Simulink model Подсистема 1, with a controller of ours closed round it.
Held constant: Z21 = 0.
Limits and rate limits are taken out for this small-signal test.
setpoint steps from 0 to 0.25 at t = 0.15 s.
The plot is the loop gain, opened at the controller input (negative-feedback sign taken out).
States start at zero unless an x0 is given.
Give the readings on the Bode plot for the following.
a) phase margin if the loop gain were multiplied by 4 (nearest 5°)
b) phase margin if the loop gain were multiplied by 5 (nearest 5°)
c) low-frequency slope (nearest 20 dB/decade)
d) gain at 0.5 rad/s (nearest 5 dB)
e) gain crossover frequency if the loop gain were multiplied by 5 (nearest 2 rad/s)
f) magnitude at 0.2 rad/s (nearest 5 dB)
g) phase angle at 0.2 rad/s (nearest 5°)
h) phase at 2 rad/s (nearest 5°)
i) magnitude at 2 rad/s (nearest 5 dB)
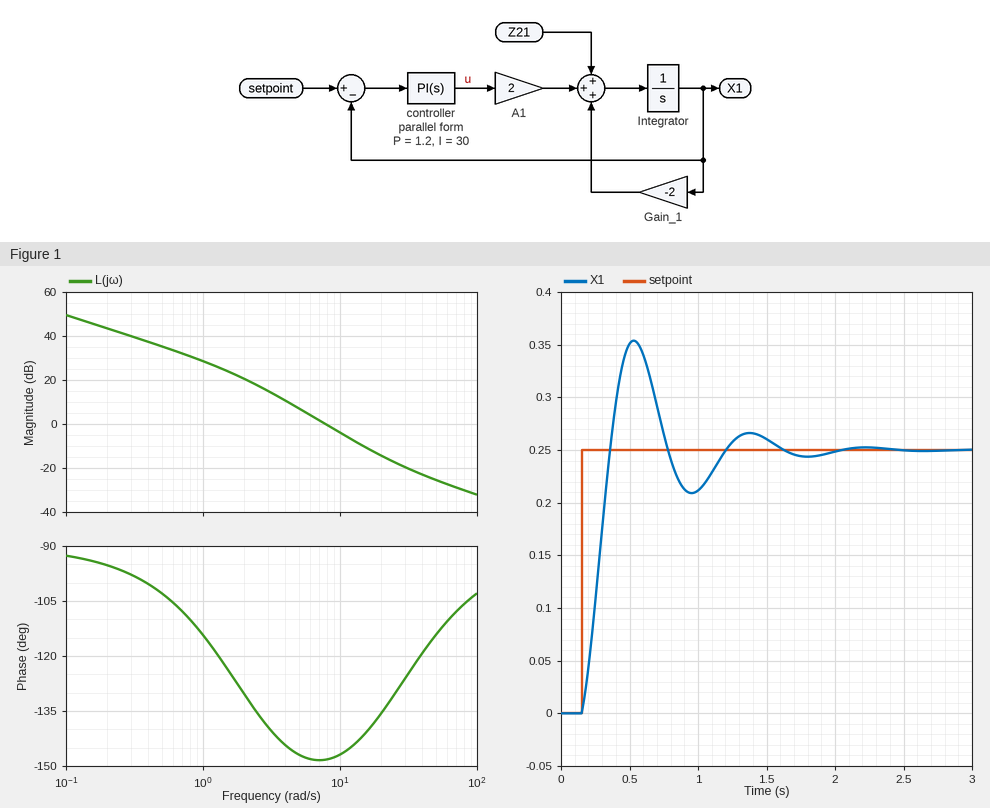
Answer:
40°
45°
-20 dB/decade
35 dB
20 rad/s
45 dB
-95°
-130°
20 dB
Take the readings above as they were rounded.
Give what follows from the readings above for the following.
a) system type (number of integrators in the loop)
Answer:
1
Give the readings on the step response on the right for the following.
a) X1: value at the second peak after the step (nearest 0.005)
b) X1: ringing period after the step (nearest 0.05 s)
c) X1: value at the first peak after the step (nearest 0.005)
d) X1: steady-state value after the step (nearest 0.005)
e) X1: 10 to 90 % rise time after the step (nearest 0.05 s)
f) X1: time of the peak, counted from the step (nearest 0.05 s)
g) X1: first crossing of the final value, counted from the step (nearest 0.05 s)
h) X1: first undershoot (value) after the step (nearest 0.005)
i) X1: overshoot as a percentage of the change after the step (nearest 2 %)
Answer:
0.265
0.85 s
0.355
0.250
0.15 s
0.40 s
0.20 s
0.210
42 %
